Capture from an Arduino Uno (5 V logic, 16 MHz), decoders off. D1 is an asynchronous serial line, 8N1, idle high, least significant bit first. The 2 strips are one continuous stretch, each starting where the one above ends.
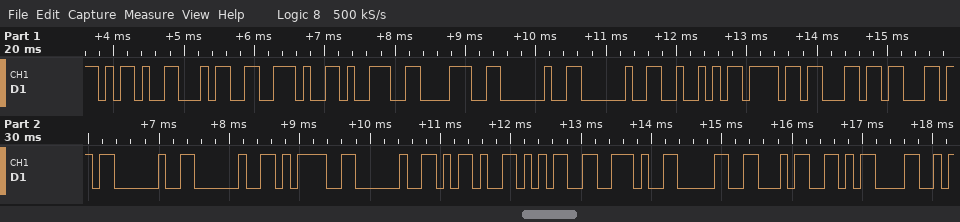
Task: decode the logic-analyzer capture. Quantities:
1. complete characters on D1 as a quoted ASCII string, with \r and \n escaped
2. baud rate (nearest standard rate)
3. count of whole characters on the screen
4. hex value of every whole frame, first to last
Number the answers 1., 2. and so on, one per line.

1. "-4.98  Roll  = -5.04\r"
2. 9600 baud
3. 21
4. 0x2D 0x34 0x2E 0x39 0x38 0x20 0x20 0x52 0x6F 0x6C 0x6C 0x20 0x20 0x3D 0x20 0x2D 0x35 0x2E 0x30 0x34 0x0D
